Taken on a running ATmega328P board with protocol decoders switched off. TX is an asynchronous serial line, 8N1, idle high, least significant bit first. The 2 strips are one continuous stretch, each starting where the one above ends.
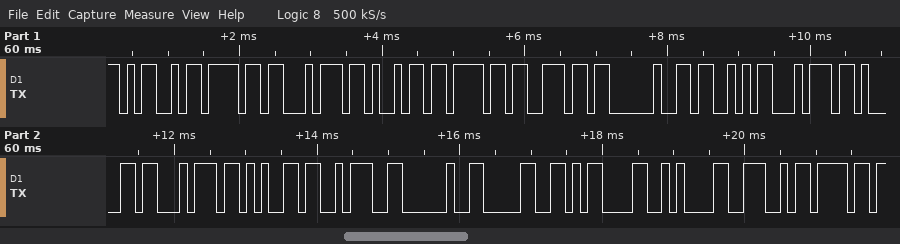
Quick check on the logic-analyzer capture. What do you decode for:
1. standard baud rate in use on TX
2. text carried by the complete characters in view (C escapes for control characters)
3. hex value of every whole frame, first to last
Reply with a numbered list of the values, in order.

1. 9600 baud
2. "Motion State: 0\r\nNo"
3. 4D 6F 74 69 6F 6E 20 53 74 61 74 65 3A 20 30 0D 0A 4E 6F
